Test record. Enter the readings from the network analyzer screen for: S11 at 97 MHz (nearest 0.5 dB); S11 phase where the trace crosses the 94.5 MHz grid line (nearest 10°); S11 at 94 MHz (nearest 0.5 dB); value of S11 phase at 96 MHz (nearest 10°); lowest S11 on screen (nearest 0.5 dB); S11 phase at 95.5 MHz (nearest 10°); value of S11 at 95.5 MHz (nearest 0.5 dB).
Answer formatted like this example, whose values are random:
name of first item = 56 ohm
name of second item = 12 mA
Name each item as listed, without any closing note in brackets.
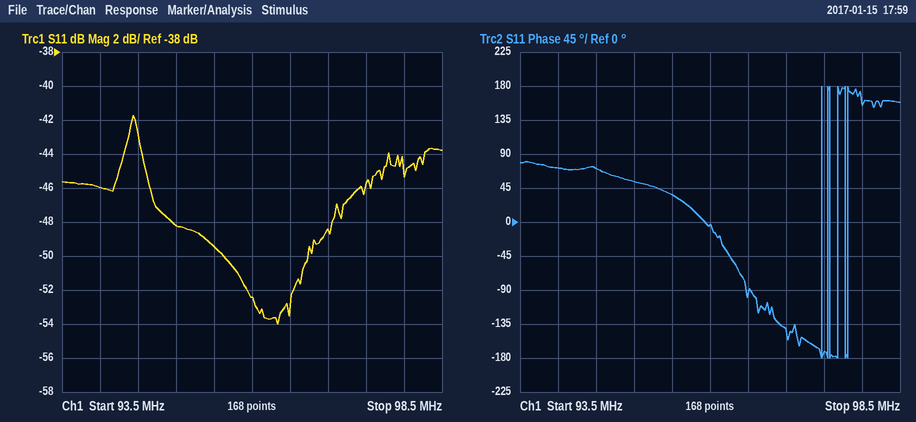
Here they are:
S11 at 97 MHz = -48.5 dB
S11 phase where the trace crosses the 94.5 MHz grid line = 70°
S11 at 94 MHz = -46.0 dB
value of S11 phase at 96 MHz = 0°
lowest S11 on screen = -54.0 dB
S11 phase at 95.5 MHz = 40°
value of S11 at 95.5 MHz = -49.5 dB
